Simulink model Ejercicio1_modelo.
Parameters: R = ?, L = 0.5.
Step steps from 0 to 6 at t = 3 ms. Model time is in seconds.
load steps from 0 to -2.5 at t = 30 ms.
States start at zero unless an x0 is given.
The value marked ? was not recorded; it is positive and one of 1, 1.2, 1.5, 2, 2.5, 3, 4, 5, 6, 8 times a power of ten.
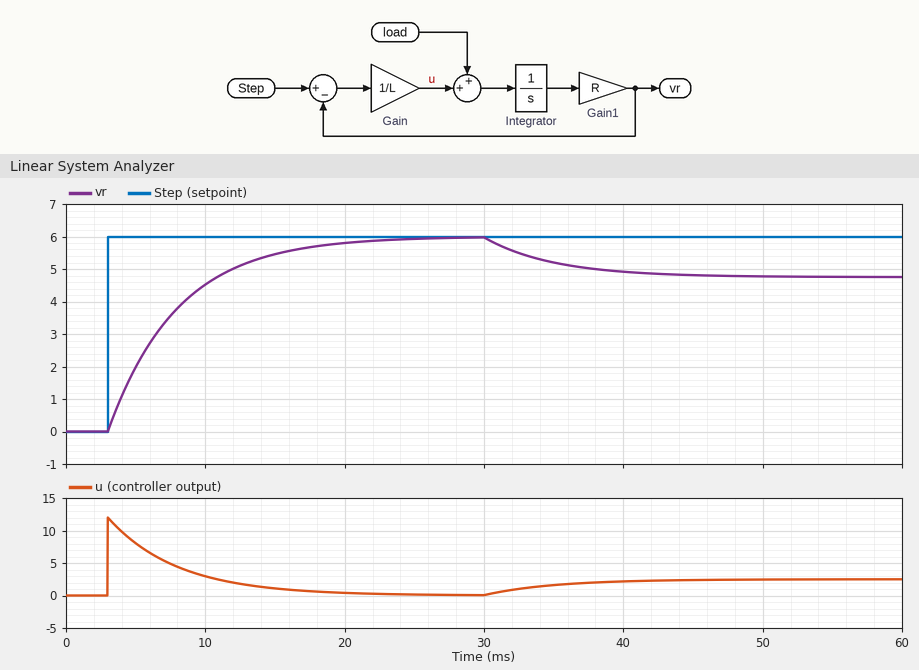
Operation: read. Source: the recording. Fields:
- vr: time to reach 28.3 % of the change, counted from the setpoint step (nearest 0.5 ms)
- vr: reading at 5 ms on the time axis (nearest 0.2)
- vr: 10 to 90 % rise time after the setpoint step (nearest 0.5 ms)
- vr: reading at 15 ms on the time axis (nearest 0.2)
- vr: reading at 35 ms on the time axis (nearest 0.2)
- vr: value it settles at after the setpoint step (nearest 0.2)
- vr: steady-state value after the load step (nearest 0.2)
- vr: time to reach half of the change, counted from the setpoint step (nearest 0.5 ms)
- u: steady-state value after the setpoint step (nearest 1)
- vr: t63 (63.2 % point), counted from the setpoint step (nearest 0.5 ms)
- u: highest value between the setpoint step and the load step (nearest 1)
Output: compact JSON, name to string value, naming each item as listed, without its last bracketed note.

{"vr: time to reach 28.3 % of the change, counted from the setpoint step": "1.5 ms", "vr: reading at 5 ms on the time axis": "2.0", "vr: 10 to 90 % rise time after the setpoint step": "11.0 ms", "vr: reading at 15 ms on the time axis": "5.4", "vr: reading at 35 ms on the time axis": "5.2", "vr: value it settles at after the setpoint step": "6.0", "vr: steady-state value after the load step": "4.8", "vr: time to reach half of the change, counted from the setpoint step": "3.5 ms", "u: steady-state value after the setpoint step": "0", "vr: t63 (63.2 % point), counted from the setpoint step": "5.0 ms", "u: highest value between the setpoint step and the load step": "12"}
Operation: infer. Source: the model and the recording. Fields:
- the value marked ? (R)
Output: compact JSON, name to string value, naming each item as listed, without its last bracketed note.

{"the value marked ?": "100"}
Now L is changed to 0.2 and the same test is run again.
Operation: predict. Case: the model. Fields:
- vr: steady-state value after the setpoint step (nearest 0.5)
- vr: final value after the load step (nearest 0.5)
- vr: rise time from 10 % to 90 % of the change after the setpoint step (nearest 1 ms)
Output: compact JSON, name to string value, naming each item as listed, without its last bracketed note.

{"vr: steady-state value after the setpoint step": "6.0", "vr: final value after the load step": "5.5", "vr: rise time from 10 % to 90 % of the change after the setpoint step": "4 ms"}
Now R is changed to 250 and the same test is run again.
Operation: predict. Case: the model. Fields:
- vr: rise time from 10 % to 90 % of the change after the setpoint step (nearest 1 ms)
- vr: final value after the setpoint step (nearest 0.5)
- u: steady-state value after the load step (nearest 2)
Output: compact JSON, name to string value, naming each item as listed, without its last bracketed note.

{"vr: rise time from 10 % to 90 % of the change after the setpoint step": "4 ms", "vr: final value after the setpoint step": "6.0", "u: steady-state value after the load step": "2"}
